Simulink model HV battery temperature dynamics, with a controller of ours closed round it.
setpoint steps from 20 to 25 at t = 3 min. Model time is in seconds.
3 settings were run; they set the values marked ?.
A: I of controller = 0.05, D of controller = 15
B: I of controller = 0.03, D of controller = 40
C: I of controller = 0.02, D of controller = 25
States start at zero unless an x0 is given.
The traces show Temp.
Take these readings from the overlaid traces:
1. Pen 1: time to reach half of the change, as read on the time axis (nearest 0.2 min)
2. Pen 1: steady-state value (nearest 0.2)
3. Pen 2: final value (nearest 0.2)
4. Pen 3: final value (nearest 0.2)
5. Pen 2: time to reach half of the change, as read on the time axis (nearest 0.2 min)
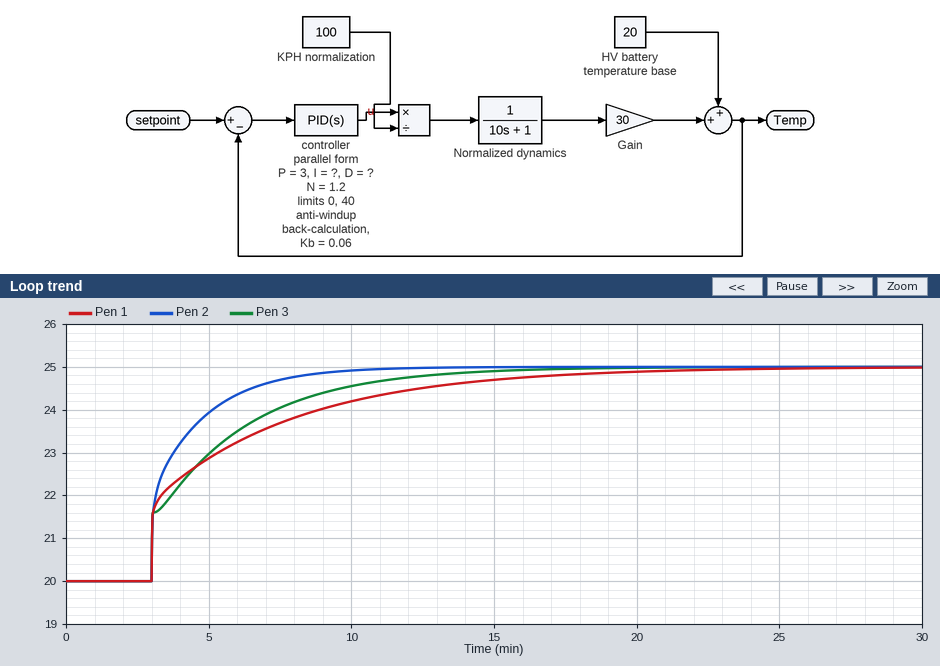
4.2 min
25.0
25.0
25.0
3.4 min
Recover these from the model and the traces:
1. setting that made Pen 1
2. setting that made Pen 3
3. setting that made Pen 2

C
B
A
